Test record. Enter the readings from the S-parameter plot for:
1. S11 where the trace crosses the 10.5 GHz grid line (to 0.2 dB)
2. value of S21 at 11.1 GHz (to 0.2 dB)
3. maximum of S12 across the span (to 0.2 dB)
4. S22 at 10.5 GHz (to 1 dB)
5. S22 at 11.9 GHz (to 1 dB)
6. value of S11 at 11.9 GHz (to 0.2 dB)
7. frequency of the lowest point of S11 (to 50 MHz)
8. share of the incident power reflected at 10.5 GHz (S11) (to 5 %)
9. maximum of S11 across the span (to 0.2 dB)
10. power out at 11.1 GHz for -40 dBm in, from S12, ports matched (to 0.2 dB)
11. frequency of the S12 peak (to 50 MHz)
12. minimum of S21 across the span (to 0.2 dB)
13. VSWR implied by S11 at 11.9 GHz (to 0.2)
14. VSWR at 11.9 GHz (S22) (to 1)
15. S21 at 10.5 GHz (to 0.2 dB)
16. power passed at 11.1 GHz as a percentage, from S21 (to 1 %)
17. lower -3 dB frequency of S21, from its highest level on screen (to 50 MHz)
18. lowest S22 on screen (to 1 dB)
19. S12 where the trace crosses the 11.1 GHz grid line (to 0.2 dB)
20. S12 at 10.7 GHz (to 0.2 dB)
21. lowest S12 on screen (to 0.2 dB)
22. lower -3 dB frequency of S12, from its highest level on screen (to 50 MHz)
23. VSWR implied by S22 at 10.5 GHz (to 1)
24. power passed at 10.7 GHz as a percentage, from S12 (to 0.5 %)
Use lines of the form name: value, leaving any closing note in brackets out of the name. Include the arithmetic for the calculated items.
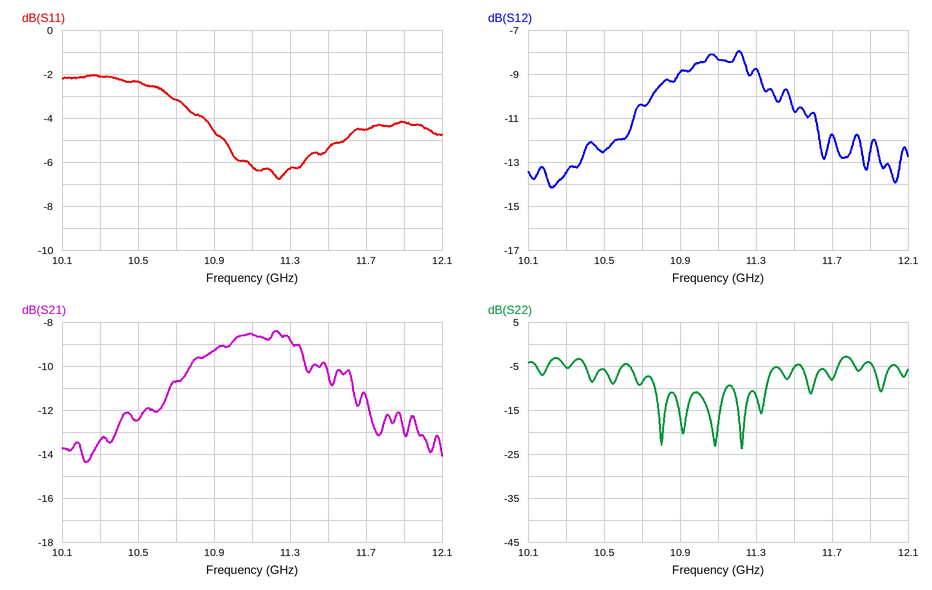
S11 where the trace crosses the 10.5 GHz grid line: -2.4 dB
value of S21 at 11.1 GHz: -8.6 dB
maximum of S12 across the span: -8.0 dB
S22 at 10.5 GHz: -6 dB
S22 at 11.9 GHz: -4 dB
value of S11 at 11.9 GHz: -4.2 dB
frequency of the lowest point of S11: 11.25 GHz
share of the incident power reflected at 10.5 GHz (S11): 10^(-2.4/10) ≈ 57.5 %, so 60 % to the nearest 5 %
maximum of S11 across the span: -2.0 dB
power out at 11.1 GHz for -40 dBm in, from S12, ports matched: -40 dBm + (-8.4 dB) = -48.4 dBm
frequency of the S12 peak: 11.20 GHz
minimum of S21 across the span: -14.4 dB
VSWR implied by S11 at 11.9 GHz: |Γ| = 10^(-4.2/20) = 0.6166; VSWR = (1 + 0.6166)/(1 − 0.6166) ≈ 4.2
VSWR at 11.9 GHz (S22): |Γ| = 10^(-4/20) = 0.6310; VSWR = (1 + 0.6310)/(1 − 0.6310) ≈ 4
S21 at 10.5 GHz: -12.4 dB
power passed at 11.1 GHz as a percentage, from S21: 10^(-8.6/10) ≈ 14 %
lower -3 dB frequency of S21, from its highest level on screen: 10.65 GHz
lowest S22 on screen: -24 dB
S12 where the trace crosses the 11.1 GHz grid line: -8.4 dB
S12 at 10.7 GHz: -10.4 dB
lowest S12 on screen: -14.2 dB
lower -3 dB frequency of S12, from its highest level on screen: 10.65 GHz
VSWR implied by S22 at 10.5 GHz: |Γ| = 10^(-6/20) = 0.5012; VSWR = (1 + 0.5012)/(1 − 0.5012) ≈ 3
power passed at 10.7 GHz as a percentage, from S12: 10^(-10.4/10) ≈ 9.12 %, so 9.0 % to the nearest 0.5 %
